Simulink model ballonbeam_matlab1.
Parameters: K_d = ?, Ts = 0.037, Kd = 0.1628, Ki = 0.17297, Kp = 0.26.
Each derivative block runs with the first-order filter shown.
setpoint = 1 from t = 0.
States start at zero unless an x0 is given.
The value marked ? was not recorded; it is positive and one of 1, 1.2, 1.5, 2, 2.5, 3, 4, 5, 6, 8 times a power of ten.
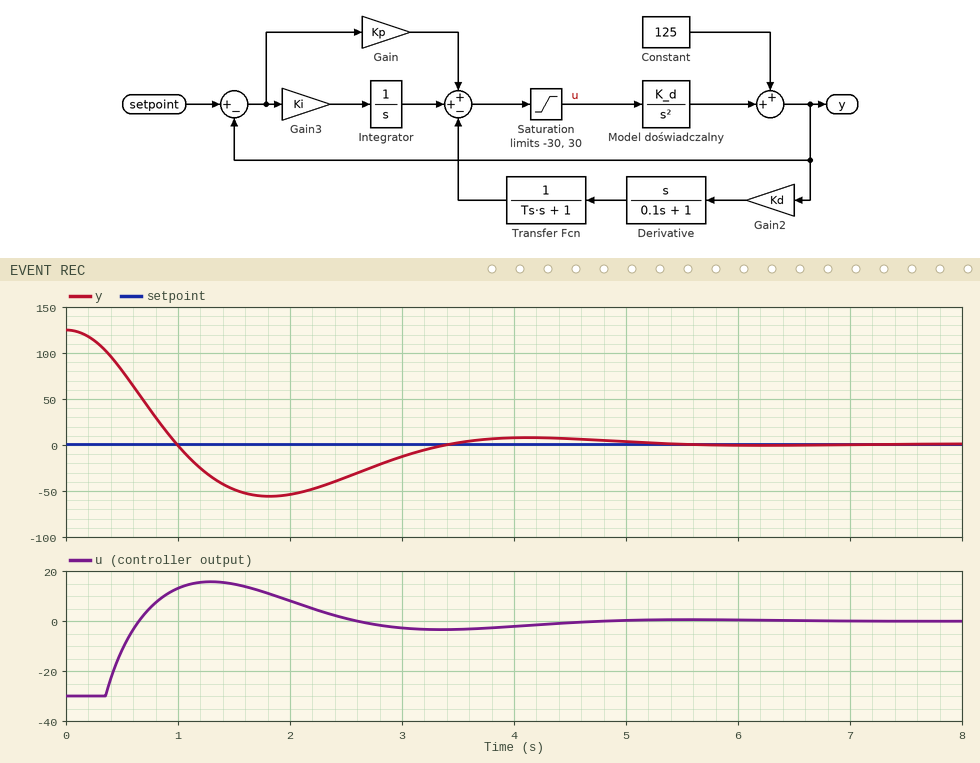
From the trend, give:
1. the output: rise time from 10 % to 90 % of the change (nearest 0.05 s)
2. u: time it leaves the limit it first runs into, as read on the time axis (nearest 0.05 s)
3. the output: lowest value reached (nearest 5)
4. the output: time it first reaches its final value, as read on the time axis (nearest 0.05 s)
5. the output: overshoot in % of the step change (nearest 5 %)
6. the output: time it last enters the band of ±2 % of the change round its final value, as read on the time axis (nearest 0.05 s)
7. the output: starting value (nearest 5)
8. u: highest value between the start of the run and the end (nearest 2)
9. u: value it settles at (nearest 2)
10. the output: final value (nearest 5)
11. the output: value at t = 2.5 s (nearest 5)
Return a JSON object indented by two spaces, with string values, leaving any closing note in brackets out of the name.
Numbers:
{
  "the output: rise time from 10 % to 90 % of the change": "0.65 s",
  "u: time it leaves the limit it first runs into, as read on the time axis": "0.35 s",
  "the output: lowest value reached": "-55",
  "the output: time it first reaches its final value, as read on the time axis": "1.00 s",
  "the output: overshoot in % of the step change": "45 %",
  "the output: time it last enters the band of ±2 % of the change round its final value, as read on the time axis": "5.00 s",
  "the output: starting value": "125",
  "u: highest value between the start of the run and the end": "16",
  "u: value it settles at": "0",
  "the output: final value": "0",
  "the output: value at t = 2.5 s": "-35"
}
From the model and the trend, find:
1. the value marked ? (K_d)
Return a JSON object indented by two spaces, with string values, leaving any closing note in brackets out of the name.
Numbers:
{
  "the value marked ?": "12"
}
